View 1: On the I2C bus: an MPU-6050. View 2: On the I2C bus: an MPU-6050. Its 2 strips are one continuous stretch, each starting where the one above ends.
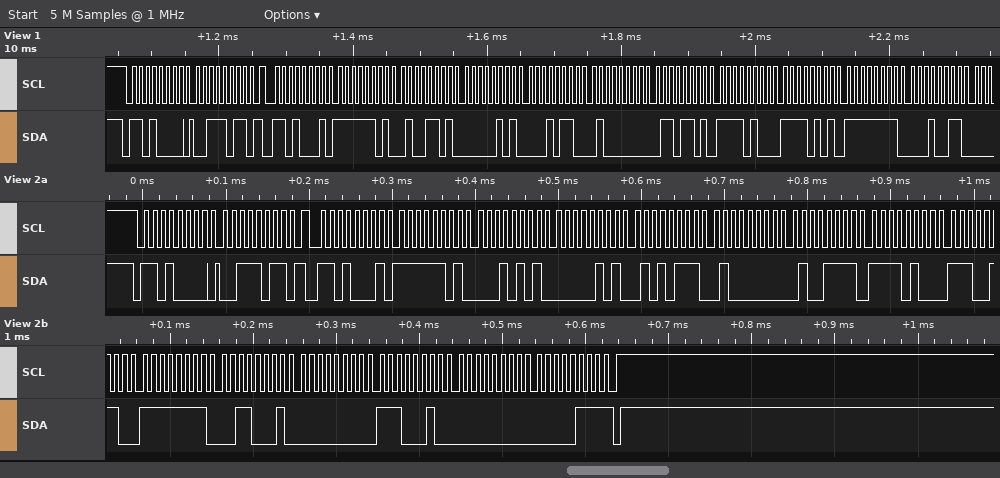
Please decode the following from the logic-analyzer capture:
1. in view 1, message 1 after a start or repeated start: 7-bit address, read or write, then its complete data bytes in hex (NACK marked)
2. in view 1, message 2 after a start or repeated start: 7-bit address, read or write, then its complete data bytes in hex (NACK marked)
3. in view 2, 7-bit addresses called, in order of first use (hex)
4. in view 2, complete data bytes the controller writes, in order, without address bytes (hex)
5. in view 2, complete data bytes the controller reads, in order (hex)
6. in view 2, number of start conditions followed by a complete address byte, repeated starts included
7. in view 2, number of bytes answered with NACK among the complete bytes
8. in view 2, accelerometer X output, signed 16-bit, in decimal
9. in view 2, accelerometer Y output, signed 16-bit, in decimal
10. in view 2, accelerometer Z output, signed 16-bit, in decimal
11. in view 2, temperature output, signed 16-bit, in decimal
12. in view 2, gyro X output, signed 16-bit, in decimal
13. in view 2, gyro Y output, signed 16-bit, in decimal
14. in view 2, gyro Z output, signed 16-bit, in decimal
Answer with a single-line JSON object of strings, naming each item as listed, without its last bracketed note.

{"in view 1, message 1 after a start or repeated start: 7-bit address, read or write, then its complete data bytes in hex": "0x68 write: 3B", "in view 1, message 2 after a start or repeated start: 7-bit address, read or write, then its complete data bytes in hex": "0x68 read: FD 4D 05 16 40 6D F4 F5 FF 13", "in view 2, 7-bit addresses called, in order of first use": "0x68", "in view 2, complete data bytes the controller writes, in order, without address bytes": "3B", "in view 2, complete data bytes the controller reads, in order": "FD 15 05 57 40 4F F4 E6 FF 31 00 E2 00 07", "in view 2, number of start conditions followed by a complete address byte, repeated starts included": "2", "in view 2, number of bytes answered with NACK among the complete bytes": "1", "in view 2, accelerometer X output, signed 16-bit, in decimal": "-747", "in view 2, accelerometer Y output, signed 16-bit, in decimal": "1367", "in view 2, accelerometer Z output, signed 16-bit, in decimal": "16463", "in view 2, temperature output, signed 16-bit, in decimal": "-2842", "in view 2, gyro X output, signed 16-bit, in decimal": "-207", "in view 2, gyro Y output, signed 16-bit, in decimal": "226", "in view 2, gyro Z output, signed 16-bit, in decimal": "7"}
